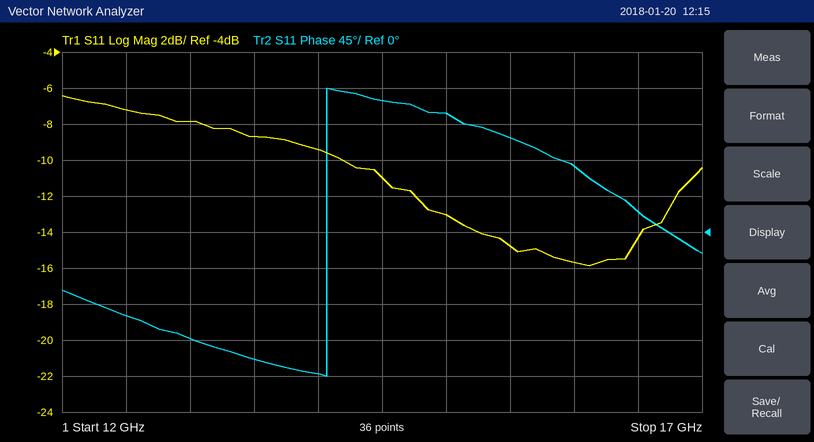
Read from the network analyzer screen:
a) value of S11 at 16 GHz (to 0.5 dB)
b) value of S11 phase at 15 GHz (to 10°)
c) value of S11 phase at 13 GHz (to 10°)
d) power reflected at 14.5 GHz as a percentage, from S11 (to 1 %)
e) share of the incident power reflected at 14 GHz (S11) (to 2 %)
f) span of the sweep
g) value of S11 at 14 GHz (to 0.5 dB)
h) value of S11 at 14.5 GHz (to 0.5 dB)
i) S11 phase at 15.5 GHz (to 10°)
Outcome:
-15.5 dB
150°
-130°
8 %
12 %
5 GHz
-9.5 dB
-11.0 dB
120°
